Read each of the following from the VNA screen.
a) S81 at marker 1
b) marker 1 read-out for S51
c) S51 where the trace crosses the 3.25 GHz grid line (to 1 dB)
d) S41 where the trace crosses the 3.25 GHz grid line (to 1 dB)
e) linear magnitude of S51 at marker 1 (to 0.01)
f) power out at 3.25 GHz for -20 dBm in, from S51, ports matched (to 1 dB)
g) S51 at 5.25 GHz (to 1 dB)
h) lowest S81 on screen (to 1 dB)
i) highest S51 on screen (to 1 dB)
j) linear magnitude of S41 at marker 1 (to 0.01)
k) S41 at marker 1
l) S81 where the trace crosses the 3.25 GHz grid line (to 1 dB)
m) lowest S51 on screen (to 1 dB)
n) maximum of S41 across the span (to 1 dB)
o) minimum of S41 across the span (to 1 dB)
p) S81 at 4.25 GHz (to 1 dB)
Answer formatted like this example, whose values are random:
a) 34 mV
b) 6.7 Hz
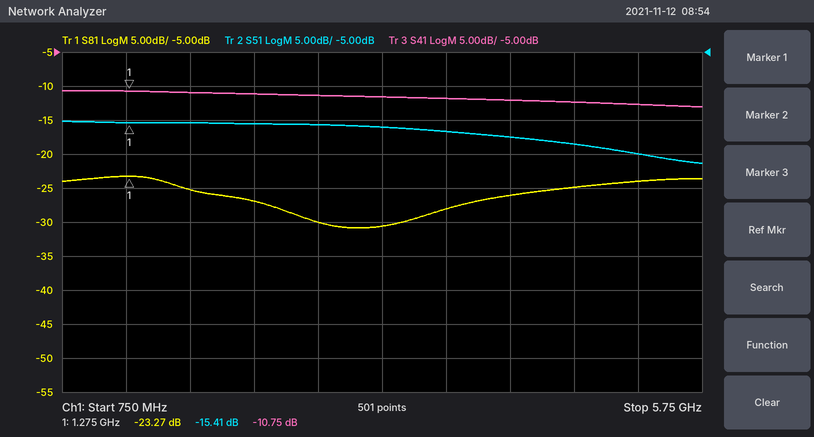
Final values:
a) -23.27 dB
b) -15.41 dB
c) -16 dB
d) -12 dB
e) 0.17
f) -36 dBm
g) -20 dB
h) -31 dB
i) -15 dB
j) 0.29
k) -10.75 dB
l) -31 dB
m) -21 dB
n) -11 dB
o) -13 dB
p) -26 dB
